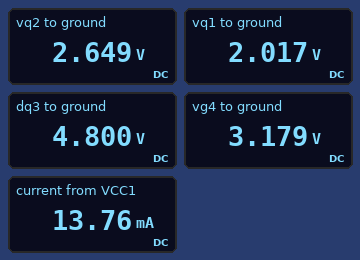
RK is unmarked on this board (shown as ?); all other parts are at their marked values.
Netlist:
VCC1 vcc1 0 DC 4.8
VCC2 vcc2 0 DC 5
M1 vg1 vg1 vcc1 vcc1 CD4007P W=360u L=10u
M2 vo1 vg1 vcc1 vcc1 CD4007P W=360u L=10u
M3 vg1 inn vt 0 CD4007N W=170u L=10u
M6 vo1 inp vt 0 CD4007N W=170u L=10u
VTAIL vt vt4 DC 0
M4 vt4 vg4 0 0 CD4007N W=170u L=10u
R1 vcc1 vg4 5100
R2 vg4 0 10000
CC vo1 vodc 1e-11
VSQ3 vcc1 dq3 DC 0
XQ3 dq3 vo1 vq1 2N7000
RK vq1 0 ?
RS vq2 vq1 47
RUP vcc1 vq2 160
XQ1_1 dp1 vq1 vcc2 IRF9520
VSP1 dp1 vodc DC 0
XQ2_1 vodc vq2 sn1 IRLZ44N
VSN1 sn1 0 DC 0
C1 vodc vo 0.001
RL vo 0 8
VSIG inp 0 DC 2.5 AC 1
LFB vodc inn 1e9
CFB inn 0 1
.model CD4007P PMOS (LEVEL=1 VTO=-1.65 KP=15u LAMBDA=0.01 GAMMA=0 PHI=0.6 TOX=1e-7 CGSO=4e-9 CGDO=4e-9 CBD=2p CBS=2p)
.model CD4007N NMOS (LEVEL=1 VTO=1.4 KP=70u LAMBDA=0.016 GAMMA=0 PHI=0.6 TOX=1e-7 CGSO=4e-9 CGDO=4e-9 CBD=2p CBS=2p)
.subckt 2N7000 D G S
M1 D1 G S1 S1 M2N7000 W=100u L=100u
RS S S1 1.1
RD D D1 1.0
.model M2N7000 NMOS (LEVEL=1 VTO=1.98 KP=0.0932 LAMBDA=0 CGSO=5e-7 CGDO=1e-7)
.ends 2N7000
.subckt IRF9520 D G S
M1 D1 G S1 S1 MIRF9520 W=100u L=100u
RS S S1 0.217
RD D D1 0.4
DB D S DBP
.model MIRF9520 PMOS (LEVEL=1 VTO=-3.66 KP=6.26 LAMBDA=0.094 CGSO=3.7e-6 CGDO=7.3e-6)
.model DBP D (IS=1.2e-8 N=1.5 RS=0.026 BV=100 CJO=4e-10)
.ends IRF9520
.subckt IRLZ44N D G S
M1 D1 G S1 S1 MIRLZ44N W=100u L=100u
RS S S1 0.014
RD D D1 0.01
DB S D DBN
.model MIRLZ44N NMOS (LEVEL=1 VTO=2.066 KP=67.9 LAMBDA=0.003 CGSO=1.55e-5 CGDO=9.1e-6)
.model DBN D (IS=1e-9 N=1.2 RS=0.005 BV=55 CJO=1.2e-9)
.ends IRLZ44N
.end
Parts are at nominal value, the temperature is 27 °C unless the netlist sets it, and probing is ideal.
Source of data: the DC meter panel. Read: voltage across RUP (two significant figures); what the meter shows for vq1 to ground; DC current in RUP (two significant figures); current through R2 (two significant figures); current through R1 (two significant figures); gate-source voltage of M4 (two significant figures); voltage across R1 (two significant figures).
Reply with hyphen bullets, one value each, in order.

- 2.2 V
- 2.017 V
- 13 mA
- 320 µA
- 320 µA
- 3.2 V
- 1.6 V
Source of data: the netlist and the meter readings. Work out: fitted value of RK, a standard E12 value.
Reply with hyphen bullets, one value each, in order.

- 150 Ω
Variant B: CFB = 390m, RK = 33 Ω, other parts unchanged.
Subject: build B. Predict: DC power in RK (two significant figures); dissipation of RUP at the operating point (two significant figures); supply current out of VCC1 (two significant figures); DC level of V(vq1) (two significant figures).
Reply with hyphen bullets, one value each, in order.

- 50 mW
- 46 mW
- 40 mA
- 1.3 V
